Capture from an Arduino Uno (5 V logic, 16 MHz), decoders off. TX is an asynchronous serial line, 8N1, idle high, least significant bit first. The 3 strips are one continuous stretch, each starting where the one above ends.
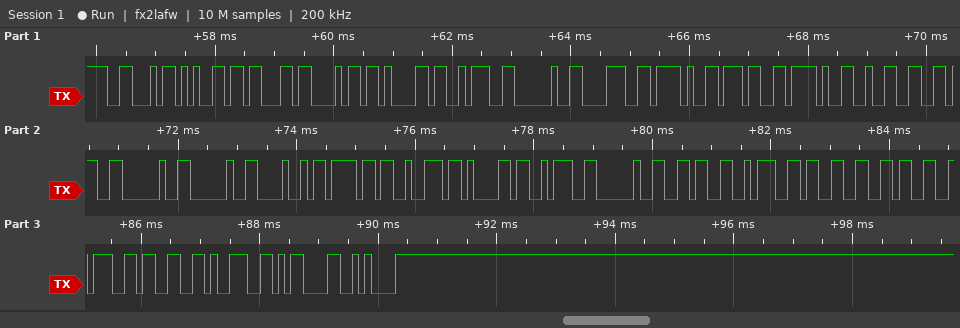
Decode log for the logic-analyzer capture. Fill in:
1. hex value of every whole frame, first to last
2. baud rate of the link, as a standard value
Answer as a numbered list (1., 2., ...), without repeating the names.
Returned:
1. 46 65 63 68 61 3A 20 38 2F 37 2F 32 36 20 20 48 6F 72 61 3A 20 36 3A 33 36 3A 33 39 0D 0A
2. 9600 baud
